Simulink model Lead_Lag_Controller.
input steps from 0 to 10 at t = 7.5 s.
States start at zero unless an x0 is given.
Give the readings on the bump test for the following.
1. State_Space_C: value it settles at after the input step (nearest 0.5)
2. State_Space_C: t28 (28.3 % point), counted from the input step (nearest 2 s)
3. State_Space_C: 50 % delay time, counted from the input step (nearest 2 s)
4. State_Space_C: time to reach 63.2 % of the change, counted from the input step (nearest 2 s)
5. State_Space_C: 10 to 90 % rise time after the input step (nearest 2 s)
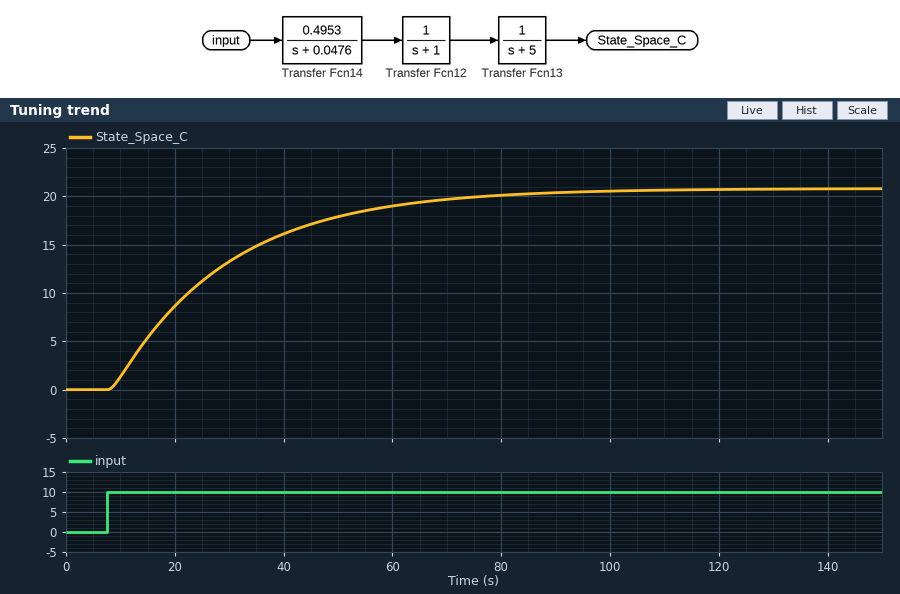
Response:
21.0
8 s
16 s
22 s
46 s
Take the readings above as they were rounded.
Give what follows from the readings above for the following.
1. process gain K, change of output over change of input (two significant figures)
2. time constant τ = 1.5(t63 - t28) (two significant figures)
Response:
2.1
21 s
